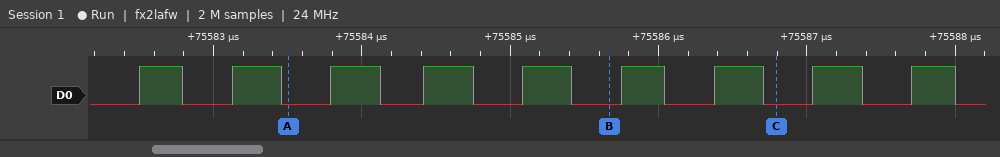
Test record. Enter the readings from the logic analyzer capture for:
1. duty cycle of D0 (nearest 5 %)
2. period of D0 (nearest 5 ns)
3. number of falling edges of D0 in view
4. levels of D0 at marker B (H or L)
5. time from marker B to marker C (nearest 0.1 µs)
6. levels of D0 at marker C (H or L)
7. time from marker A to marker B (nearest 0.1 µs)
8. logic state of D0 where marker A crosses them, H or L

50 %
650 ns
9
D0=L
1.1 µs
D0=L
2.2 µs
D0=L
